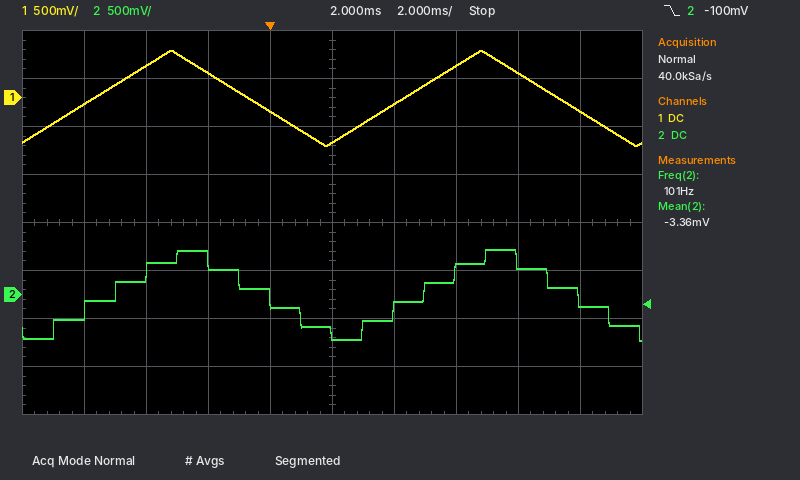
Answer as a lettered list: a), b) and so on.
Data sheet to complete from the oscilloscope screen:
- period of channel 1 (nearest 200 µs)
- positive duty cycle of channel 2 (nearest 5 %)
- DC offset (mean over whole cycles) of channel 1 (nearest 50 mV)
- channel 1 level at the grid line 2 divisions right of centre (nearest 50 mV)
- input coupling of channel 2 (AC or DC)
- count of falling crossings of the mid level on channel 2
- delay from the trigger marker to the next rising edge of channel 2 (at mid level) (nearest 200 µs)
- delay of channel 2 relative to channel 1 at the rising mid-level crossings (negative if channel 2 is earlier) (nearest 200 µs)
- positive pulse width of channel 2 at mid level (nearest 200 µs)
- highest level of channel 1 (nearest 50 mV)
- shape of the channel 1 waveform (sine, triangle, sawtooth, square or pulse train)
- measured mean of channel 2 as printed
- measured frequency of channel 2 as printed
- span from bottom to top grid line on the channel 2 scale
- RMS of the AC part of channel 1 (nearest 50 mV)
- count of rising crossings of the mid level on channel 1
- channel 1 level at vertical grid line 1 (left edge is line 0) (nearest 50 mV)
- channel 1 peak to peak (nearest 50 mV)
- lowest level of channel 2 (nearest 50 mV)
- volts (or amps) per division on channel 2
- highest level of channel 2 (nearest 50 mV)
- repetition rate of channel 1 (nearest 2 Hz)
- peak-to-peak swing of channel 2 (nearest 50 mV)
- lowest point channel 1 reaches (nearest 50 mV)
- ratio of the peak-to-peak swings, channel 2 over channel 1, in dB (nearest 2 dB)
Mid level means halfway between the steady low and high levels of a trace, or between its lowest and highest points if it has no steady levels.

a) 10.0 ms
b) 50 %
c) 0 mV
d) 350 mV
e) DC
f) 2
g) 5.0 ms
h) +600 µs
i) 5.0 ms
j) 500 mV
k) triangle
l) -3.36 mV
m) 101 Hz
n) 4 V
o) 300 mV
p) 2
q) -50 mV
r) 1.00 V
s) -500 mV
t) 500 mV
u) 450 mV
v) 100 Hz
w) 950 mV
x) -500 mV
y) 0 dB
